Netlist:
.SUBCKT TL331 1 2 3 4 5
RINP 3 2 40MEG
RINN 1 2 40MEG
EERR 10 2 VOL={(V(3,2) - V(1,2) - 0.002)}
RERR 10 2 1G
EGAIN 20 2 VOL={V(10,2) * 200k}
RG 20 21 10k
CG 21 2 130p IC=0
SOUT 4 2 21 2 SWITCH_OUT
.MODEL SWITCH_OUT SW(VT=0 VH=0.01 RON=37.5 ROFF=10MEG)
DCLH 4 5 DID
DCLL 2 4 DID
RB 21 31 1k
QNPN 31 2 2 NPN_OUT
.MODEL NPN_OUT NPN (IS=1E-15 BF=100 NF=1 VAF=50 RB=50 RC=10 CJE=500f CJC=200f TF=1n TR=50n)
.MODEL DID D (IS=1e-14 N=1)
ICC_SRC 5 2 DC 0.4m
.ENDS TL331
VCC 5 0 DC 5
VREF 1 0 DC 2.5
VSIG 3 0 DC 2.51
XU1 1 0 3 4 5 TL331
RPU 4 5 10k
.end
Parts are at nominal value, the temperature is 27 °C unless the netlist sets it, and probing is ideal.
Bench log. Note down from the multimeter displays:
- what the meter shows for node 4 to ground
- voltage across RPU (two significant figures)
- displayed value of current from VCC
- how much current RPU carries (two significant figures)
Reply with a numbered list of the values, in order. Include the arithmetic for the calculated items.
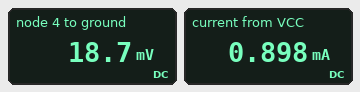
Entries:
1. 18.7 mV
2. 5 V - 18.7 mV = 5.0 V
3. 0.898 mA
4. (5 V - 18.7 mV) / 10 kΩ = 500 µA
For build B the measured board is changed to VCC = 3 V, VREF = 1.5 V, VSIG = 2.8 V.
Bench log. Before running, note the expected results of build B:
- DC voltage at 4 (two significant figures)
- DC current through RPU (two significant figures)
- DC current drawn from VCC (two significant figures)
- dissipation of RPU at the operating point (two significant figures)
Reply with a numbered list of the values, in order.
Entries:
1. 11 mV
2. 300 µA
3. 700 µA
4. 890 µW
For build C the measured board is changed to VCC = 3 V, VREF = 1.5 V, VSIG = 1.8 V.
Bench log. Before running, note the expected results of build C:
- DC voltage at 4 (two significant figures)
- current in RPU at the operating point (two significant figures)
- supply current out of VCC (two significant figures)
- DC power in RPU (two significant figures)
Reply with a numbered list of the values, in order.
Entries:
1. 11 mV
2. 300 µA
3. 700 µA
4. 890 µW
